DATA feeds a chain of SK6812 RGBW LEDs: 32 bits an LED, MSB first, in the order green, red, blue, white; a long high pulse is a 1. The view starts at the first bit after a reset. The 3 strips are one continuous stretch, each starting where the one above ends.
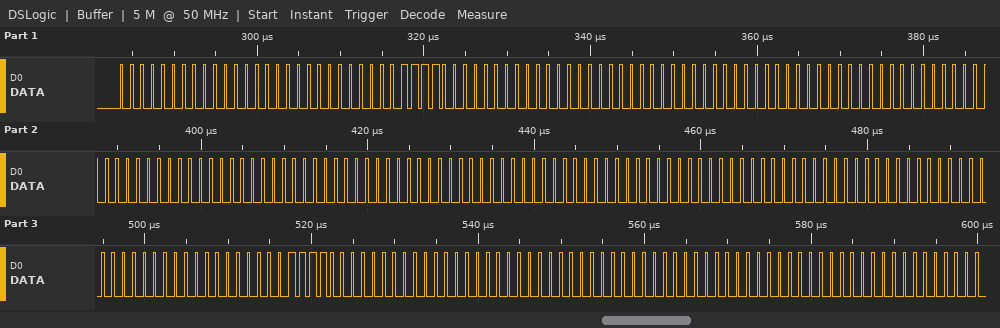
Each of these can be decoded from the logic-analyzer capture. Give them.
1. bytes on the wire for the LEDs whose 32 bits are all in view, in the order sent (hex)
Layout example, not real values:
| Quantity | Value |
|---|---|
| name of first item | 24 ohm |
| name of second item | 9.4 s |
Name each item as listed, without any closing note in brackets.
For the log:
| Quantity | Value |
|---|---|
| bytes on the wire for the LEDs whose 32 bits are all in view, in the order sent | 00 00 00 1E 00 00 00 00 00 00 00 00 00 00 00 00 00 00 00 00 00 00 00 1E 00 00 00 00 |
